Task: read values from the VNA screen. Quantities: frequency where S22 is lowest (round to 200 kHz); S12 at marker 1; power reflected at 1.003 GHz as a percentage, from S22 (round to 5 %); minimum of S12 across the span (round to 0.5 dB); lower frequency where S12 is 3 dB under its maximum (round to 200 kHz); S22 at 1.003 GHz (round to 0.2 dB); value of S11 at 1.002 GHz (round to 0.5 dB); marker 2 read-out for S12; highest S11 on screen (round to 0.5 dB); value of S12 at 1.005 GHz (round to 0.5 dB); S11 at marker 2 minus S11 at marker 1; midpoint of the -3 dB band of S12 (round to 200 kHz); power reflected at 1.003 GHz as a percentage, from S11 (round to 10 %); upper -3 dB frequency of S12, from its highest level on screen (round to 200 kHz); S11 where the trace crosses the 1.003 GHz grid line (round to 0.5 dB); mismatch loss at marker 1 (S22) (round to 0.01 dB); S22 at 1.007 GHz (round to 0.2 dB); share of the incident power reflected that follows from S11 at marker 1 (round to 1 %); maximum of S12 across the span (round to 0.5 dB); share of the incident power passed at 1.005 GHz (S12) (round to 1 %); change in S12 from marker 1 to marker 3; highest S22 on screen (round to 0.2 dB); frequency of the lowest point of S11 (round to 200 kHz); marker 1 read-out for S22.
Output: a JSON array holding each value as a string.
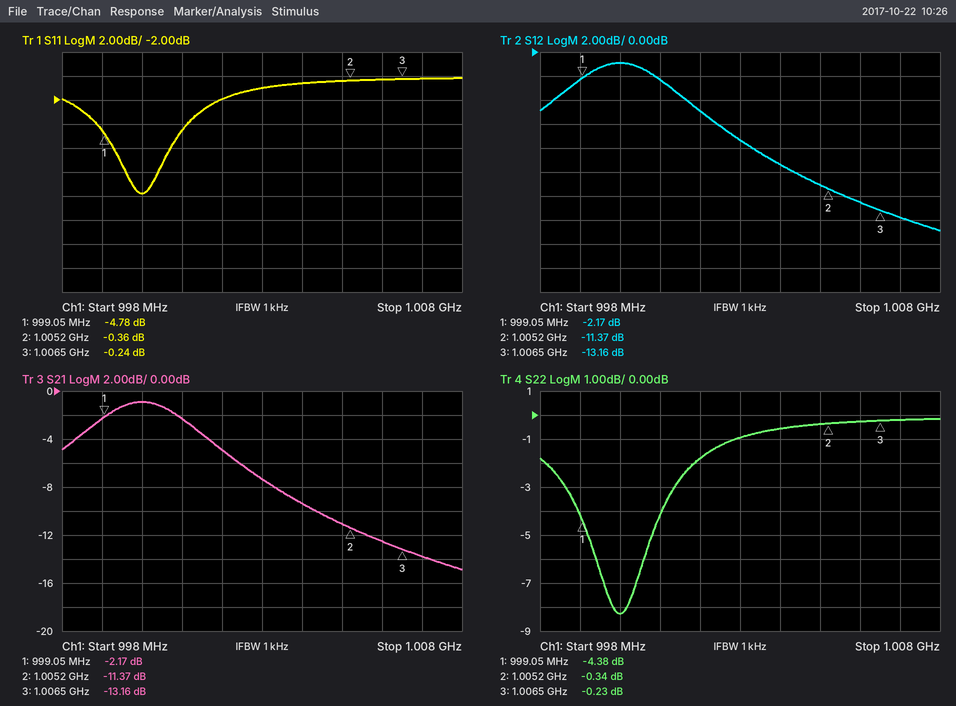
["1.0000 GHz", "-2.17 dB", "80 %", "-15.0 dB", "998.4 MHz", "-1.0 dB", "-2.0 dB", "-11.37 dB", "0.0 dB", "-11.0 dB", "4.42 dB", "1.0000 GHz", "80 %", "1.0016 GHz", "-1.0 dB", "1.97 dB", "-0.2 dB", "33 %", "-1.0 dB", "8 %", "-10.99 dB", "-0.2 dB", "1.0000 GHz", "-4.38 dB"]
